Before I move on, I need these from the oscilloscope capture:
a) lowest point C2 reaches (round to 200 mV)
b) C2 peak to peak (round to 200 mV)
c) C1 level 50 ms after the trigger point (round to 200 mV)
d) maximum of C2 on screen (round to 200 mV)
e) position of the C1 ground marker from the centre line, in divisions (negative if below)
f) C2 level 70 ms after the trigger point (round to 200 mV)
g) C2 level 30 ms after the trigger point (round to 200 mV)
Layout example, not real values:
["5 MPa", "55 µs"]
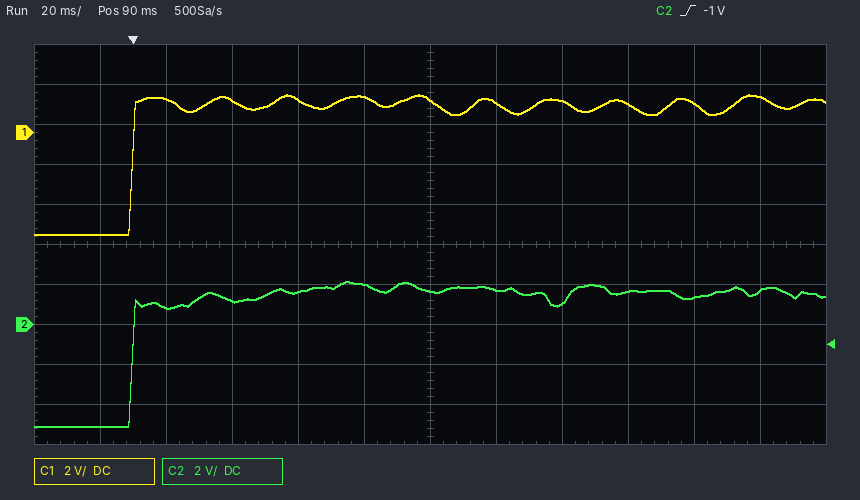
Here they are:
["-5.0 V", "7.2 V", "1.6 V", "2.2 V", "+2.8 div", "2.0 V", "1.2 V"]
